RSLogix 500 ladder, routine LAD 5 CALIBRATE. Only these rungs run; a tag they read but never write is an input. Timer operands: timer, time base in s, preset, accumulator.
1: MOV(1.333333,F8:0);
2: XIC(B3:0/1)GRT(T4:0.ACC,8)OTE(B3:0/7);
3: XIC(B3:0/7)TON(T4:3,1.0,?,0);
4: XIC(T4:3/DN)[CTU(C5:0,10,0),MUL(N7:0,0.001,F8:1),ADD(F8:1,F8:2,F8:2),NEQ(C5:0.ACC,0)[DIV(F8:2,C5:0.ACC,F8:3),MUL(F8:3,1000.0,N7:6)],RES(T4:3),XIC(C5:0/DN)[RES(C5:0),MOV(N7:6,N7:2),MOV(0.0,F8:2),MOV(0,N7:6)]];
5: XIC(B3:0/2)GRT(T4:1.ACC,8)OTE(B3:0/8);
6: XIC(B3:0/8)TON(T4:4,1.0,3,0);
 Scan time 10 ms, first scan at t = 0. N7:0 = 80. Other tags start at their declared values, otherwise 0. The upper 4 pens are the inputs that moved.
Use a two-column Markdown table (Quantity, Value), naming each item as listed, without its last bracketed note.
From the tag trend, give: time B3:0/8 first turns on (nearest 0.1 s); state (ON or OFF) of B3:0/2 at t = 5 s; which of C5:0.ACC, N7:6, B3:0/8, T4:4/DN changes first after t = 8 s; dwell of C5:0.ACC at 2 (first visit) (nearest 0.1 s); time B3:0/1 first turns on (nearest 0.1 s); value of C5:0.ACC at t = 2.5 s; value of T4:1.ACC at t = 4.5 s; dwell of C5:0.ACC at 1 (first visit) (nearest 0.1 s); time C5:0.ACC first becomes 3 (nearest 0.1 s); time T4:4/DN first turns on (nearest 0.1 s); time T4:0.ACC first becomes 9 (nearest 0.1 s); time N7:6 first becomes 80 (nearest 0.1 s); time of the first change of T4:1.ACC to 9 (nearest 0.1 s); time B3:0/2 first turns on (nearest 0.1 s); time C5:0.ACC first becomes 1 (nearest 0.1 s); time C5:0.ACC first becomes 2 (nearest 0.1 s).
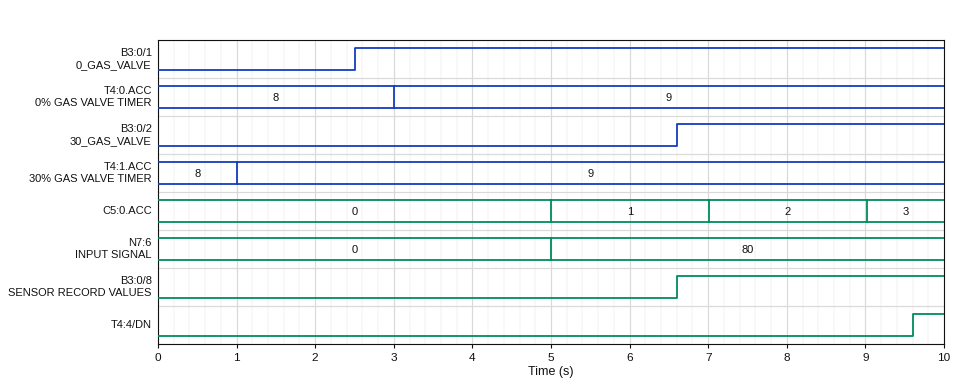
| Quantity | Value |
|---|---|
| time B3:0/8 first turns on | 6.6 s |
| state (ON or OFF) of B3:0/2 at t = 5 s | OFF |
| which of C5:0.ACC, N7:6, B3:0/8, T4:4/DN changes first after t = 8 s | C5:0.ACC |
| dwell of C5:0.ACC at 2 (first visit) | 2.0 s |
| time B3:0/1 first turns on | 2.5 s |
| value of C5:0.ACC at t = 2.5 s | 0 |
| value of T4:1.ACC at t = 4.5 s | 9 |
| dwell of C5:0.ACC at 1 (first visit) | 2.0 s |
| time C5:0.ACC first becomes 3 | 9.0 s |
| time T4:4/DN first turns on | 9.6 s |
| time T4:0.ACC first becomes 9 | 3.0 s |
| time N7:6 first becomes 80 | 5.0 s |
| time of the first change of T4:1.ACC to 9 | 1.0 s |
| time B3:0/2 first turns on | 6.6 s |
| time C5:0.ACC first becomes 1 | 5.0 s |
| time C5:0.ACC first becomes 2 | 7.0 s |
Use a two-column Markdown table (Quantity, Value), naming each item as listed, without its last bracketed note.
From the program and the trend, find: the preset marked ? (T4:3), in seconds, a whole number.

| Quantity | Value |
|---|---|
| the preset marked ? (T4:3), in seconds, a whole number | 2 s |
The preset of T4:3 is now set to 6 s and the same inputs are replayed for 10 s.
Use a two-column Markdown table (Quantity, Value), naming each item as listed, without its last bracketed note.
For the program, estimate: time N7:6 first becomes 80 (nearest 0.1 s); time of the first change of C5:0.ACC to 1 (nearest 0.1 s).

| Quantity | Value |
|---|---|
| time N7:6 first becomes 80 | 9.0 s |
| time of the first change of C5:0.ACC to 1 | 9.0 s |
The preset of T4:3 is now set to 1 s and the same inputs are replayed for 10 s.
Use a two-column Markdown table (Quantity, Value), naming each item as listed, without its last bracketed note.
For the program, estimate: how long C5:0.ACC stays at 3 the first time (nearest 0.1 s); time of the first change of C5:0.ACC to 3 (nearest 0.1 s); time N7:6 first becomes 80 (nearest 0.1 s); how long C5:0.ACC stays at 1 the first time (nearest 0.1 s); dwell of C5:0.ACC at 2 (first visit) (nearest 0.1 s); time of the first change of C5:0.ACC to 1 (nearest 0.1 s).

| Quantity | Value |
|---|---|
| how long C5:0.ACC stays at 3 the first time | 1.0 s |
| time of the first change of C5:0.ACC to 3 | 6.0 s |
| time N7:6 first becomes 80 | 4.0 s |
| how long C5:0.ACC stays at 1 the first time | 1.0 s |
| dwell of C5:0.ACC at 2 (first visit) | 1.0 s |
| time of the first change of C5:0.ACC to 1 | 4.0 s |
